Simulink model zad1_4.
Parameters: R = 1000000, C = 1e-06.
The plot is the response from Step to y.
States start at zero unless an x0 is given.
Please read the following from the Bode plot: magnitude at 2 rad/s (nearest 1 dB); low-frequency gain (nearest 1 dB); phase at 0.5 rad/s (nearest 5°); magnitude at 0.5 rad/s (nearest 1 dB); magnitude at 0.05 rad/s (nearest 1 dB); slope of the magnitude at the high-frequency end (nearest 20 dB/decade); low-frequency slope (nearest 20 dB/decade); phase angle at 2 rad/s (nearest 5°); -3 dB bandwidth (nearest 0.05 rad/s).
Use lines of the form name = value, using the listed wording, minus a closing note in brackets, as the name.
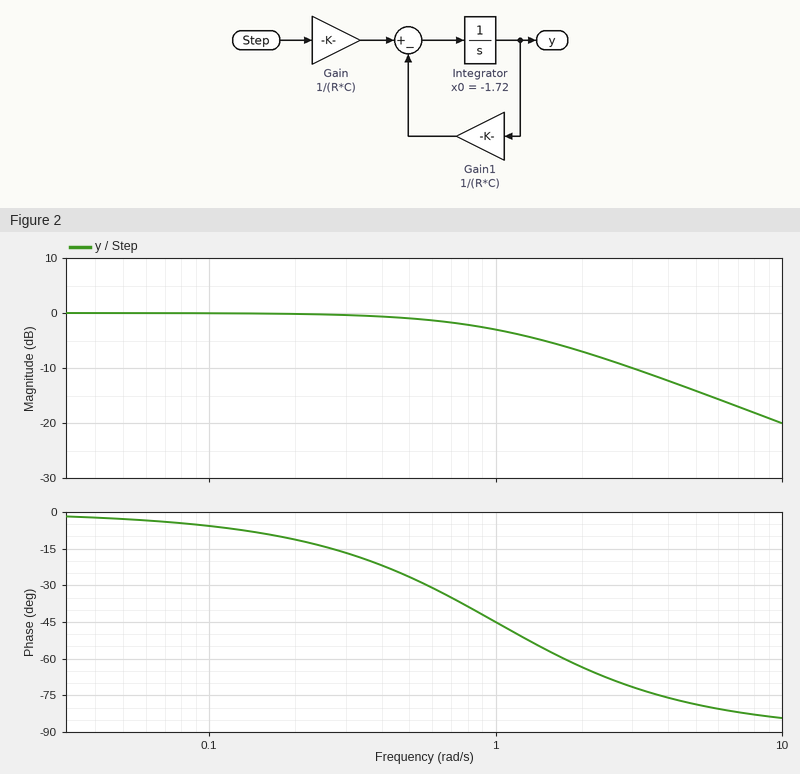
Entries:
magnitude at 2 rad/s = -7 dB
low-frequency gain = 0 dB
phase at 0.5 rad/s = -25°
magnitude at 0.5 rad/s = -1 dB
magnitude at 0.05 rad/s = 0 dB
slope of the magnitude at the high-frequency end = -20 dB/decade
low-frequency slope = 0 dB/decade
phase angle at 2 rad/s = -65°
-3 dB bandwidth = 1.00 rad/s
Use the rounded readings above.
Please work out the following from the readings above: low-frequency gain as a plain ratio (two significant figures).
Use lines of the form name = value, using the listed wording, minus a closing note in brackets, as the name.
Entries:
low-frequency gain as a plain ratio = 1.0
